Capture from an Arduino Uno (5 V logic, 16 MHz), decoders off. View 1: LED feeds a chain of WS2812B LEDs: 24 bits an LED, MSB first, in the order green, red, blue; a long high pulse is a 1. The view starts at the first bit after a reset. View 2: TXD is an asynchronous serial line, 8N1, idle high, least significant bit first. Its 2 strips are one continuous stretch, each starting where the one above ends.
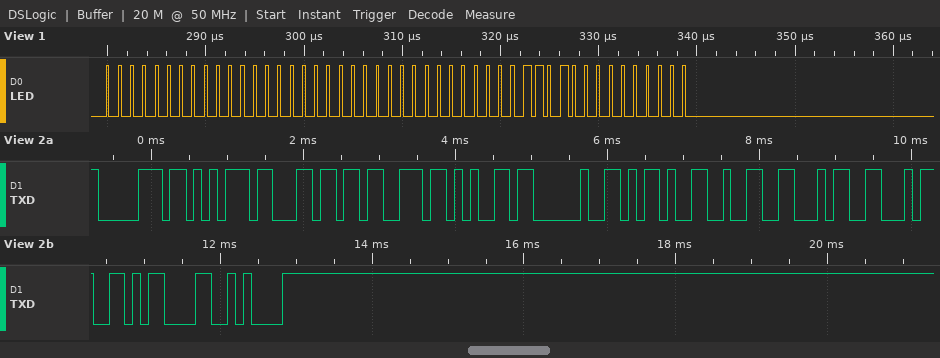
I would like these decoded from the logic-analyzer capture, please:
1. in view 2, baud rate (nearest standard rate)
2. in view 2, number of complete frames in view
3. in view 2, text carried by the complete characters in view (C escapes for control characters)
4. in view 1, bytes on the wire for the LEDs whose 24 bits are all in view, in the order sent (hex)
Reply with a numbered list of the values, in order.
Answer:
1. 9600 baud
2. 12
3. "pulse -244\r\n"
4. 00 00 00 00 34 00
